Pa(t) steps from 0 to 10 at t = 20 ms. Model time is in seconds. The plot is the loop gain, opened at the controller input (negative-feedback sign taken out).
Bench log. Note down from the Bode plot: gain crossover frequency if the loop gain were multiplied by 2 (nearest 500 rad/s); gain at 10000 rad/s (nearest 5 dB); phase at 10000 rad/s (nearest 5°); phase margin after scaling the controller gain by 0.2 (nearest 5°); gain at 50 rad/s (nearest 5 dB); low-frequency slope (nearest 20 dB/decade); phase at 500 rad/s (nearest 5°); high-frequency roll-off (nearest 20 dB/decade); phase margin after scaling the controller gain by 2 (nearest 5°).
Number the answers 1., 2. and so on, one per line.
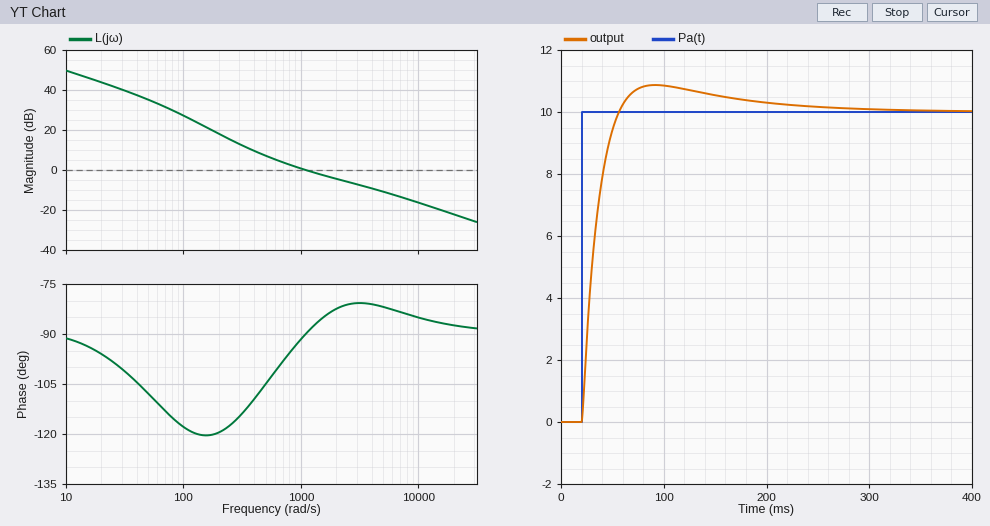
1. 2500 rad/s
2. -15 dB
3. -85°
4. 65°
5. 35 dB
6. -20 dB/decade
7. -105°
8. -20 dB/decade
9. 100°
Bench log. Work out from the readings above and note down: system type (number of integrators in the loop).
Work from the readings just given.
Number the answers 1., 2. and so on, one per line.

1. 1
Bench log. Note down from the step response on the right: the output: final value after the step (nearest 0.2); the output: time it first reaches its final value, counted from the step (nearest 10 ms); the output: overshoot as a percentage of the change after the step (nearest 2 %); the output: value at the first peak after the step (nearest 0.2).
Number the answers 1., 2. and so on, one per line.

1. 10.0
2. 40 ms
3. 8 %
4. 10.8
